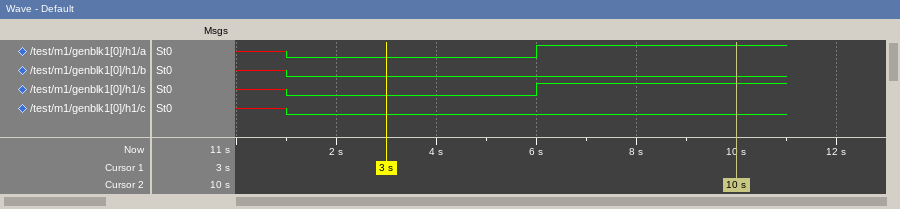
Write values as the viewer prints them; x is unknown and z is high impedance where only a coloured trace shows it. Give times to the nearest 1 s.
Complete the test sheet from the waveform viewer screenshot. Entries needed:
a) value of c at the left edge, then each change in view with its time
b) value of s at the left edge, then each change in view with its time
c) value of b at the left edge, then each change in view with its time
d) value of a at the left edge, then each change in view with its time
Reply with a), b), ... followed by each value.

a) x, 0 at 1 s
b) x, 0 at 1 s, 1 at 6 s
c) x, 0 at 1 s
d) x, 0 at 1 s, 1 at 6 s
